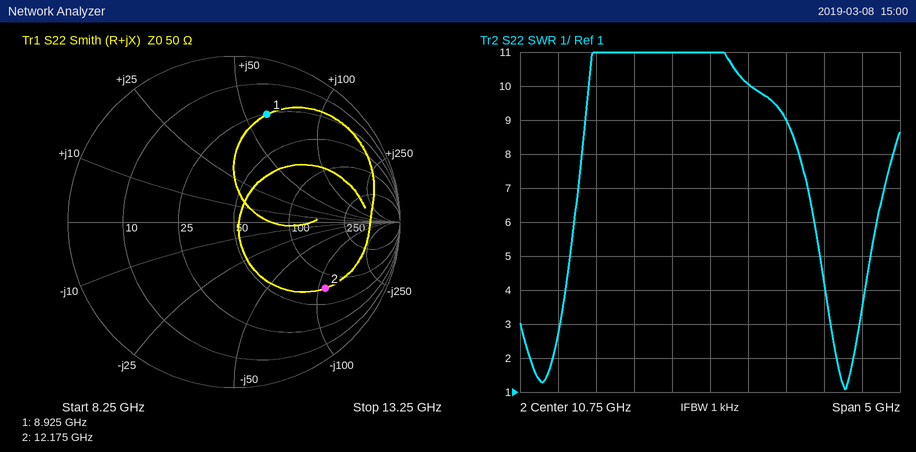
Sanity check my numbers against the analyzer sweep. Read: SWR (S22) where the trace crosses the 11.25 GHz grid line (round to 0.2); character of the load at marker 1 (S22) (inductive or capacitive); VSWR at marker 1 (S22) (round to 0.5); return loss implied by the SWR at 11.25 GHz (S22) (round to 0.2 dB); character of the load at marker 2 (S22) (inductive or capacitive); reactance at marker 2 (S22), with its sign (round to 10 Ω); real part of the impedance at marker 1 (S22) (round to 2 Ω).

10.0
inductive
5.0
1.8 dB
capacitive
-110 Ω
26 Ω
